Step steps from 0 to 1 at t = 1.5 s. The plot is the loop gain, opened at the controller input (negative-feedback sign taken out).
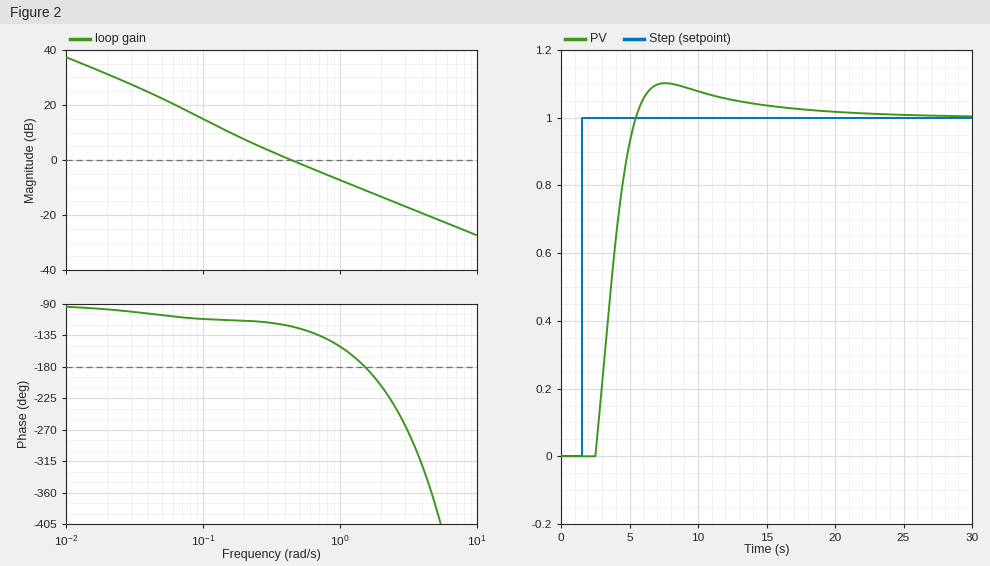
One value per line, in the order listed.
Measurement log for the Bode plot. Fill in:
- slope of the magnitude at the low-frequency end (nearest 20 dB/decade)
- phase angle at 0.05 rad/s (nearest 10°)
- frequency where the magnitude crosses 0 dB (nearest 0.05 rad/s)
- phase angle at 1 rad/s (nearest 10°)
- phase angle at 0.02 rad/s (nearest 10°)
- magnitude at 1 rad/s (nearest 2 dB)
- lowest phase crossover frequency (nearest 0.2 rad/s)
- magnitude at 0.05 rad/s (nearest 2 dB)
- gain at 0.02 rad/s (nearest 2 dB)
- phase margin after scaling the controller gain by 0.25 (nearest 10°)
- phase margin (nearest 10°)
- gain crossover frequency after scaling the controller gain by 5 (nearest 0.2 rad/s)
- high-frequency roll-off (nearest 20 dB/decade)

-20 dB/decade
-110°
0.45 rad/s
-150°
-100°
-8 dB
1.6 rad/s
22 dB
32 dB
70°
60°
2.2 rad/s
-20 dB/decade
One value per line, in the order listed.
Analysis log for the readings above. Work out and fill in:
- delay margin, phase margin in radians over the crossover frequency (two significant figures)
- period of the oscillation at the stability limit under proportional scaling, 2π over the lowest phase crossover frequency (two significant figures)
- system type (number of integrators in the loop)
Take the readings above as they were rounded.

2.3 s
3.9 s
1
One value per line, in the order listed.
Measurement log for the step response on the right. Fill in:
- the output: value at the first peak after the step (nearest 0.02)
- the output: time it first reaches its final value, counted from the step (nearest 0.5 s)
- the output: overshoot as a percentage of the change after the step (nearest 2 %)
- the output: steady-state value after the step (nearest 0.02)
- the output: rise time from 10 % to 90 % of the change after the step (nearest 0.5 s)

1.10
4.0 s
10 %
1.00
2.0 s
